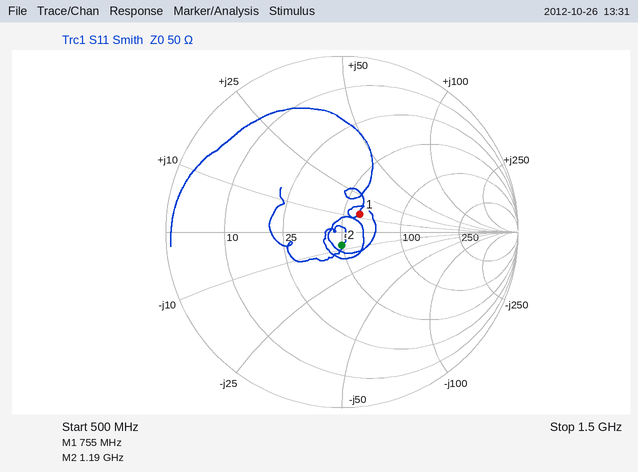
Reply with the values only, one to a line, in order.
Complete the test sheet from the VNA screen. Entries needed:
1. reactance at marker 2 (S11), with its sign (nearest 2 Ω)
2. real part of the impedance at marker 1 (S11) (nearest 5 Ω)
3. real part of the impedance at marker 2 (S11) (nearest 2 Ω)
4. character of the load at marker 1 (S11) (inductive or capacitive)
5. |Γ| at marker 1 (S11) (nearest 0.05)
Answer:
-8 Ω
60 Ω
50 Ω
inductive
0.15
